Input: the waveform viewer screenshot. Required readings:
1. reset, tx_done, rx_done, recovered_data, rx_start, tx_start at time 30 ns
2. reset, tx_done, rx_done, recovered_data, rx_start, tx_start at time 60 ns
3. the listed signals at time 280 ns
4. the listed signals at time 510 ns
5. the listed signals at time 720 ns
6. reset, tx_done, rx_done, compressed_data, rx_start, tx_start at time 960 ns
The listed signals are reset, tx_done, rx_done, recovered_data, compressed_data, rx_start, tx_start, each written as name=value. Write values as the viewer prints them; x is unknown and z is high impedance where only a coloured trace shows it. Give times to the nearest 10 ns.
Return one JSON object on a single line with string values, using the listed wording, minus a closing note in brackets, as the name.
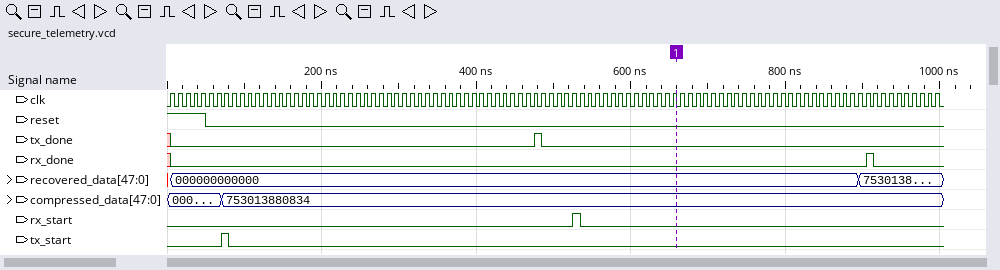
{"reset, tx_done, rx_done, recovered_data, rx_start, tx_start at time 30 ns": "reset=1, tx_done=0, rx_done=0, recovered_data=000000000000, rx_start=0, tx_start=0", "reset, tx_done, rx_done, recovered_data, rx_start, tx_start at time 60 ns": "reset=0, tx_done=0, rx_done=0, recovered_data=000000000000, rx_start=0, tx_start=0", "the listed signals at time 280 ns": "reset=0, tx_done=0, rx_done=0, recovered_data=000000000000, compressed_data=753013880834, rx_start=0, tx_start=0", "the listed signals at time 510 ns": "reset=0, tx_done=0, rx_done=0, recovered_data=000000000000, compressed_data=753013880834, rx_start=0, tx_start=0", "the listed signals at time 720 ns": "reset=0, tx_done=0, rx_done=0, recovered_data=000000000000, compressed_data=753013880834, rx_start=0, tx_start=0", "reset, tx_done, rx_done, compressed_data, rx_start, tx_start at time 960 ns": "reset=0, tx_done=0, rx_done=0, compressed_data=753013880834, rx_start=0, tx_start=0"}
